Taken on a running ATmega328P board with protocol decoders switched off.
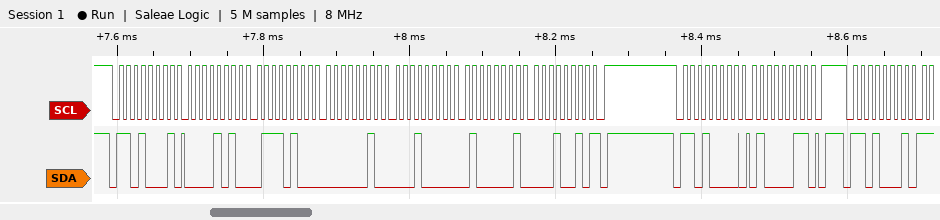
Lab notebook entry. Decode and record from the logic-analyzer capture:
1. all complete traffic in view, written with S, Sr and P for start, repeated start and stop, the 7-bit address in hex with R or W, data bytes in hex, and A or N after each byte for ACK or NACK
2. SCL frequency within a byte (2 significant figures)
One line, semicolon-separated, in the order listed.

S 68R A 0A A 74 A 02 A 10 A 41 A 12 N P S 68W A 43 A P S 68R A; 100 kHz
